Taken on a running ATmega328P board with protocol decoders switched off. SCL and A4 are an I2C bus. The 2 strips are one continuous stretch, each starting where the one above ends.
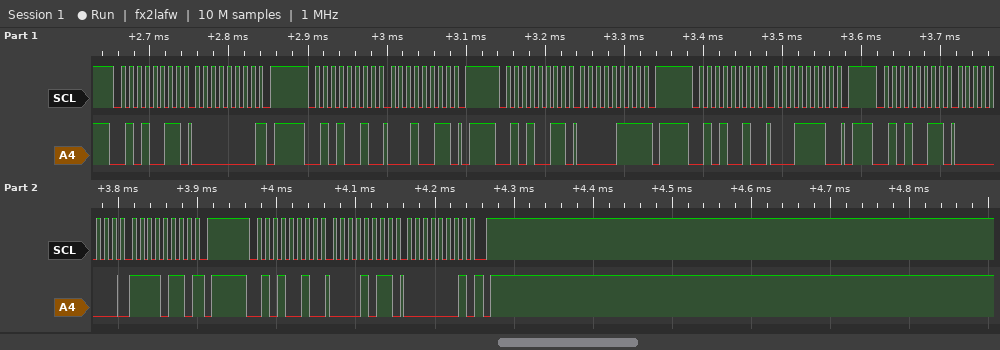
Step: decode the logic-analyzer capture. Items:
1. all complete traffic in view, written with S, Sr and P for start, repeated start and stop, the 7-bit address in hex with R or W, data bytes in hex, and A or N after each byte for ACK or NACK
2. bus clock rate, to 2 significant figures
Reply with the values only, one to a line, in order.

S 29R A 00 N P S 29W A 13 A P S 29R A 07 N P S 29W A 1E A P S 29R A 00 A F6 N P S 29W A 0B A 01 A P
100 kHz
